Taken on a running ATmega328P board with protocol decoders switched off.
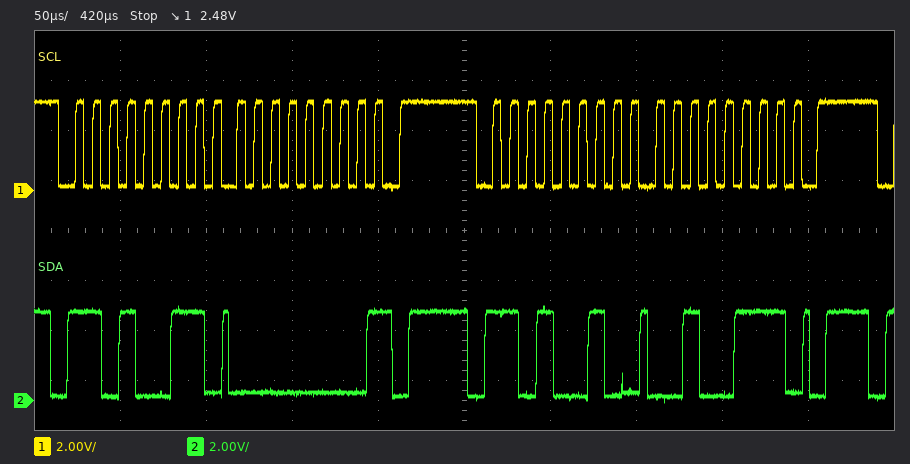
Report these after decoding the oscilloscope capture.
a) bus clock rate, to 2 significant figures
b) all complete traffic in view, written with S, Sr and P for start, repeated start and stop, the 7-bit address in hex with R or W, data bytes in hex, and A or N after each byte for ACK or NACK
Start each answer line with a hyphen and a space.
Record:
- 100 kHz
- S 69R A 00 N P S 69W A 27 A P
